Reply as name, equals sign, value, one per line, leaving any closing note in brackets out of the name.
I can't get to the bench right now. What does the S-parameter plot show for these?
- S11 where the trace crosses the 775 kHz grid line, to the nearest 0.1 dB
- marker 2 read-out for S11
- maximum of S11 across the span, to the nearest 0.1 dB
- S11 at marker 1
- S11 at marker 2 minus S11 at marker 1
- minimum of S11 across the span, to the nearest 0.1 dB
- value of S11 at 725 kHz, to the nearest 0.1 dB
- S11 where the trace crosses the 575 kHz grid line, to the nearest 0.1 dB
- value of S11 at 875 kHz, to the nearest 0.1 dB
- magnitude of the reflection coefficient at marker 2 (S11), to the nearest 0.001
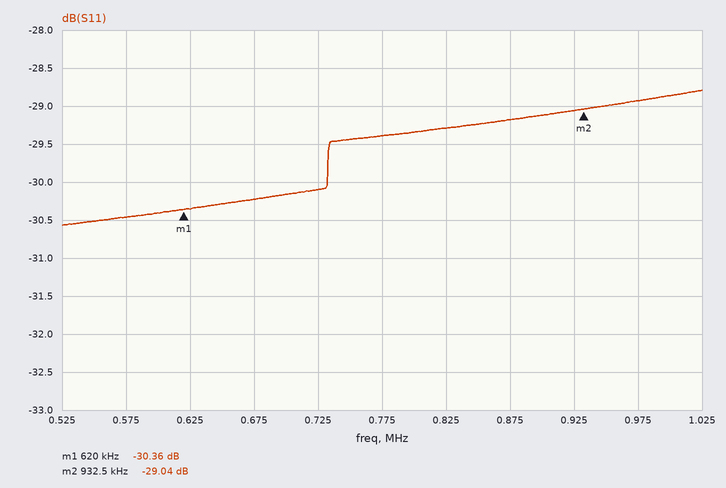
S11 where the trace crosses the 775 kHz grid line, to the nearest 0.1 dB = -29.4 dB
marker 2 read-out for S11 = -29.04 dB
maximum of S11 across the span, to the nearest 0.1 dB = -28.8 dB
S11 at marker 1 = -30.36 dB
S11 at marker 2 minus S11 at marker 1 = 1.32 dB
minimum of S11 across the span, to the nearest 0.1 dB = -30.6 dB
value of S11 at 725 kHz, to the nearest 0.1 dB = -30.1 dB
S11 where the trace crosses the 575 kHz grid line, to the nearest 0.1 dB = -30.5 dB
value of S11 at 875 kHz, to the nearest 0.1 dB = -29.2 dB
magnitude of the reflection coefficient at marker 2 (S11), to the nearest 0.001 = 0.035
